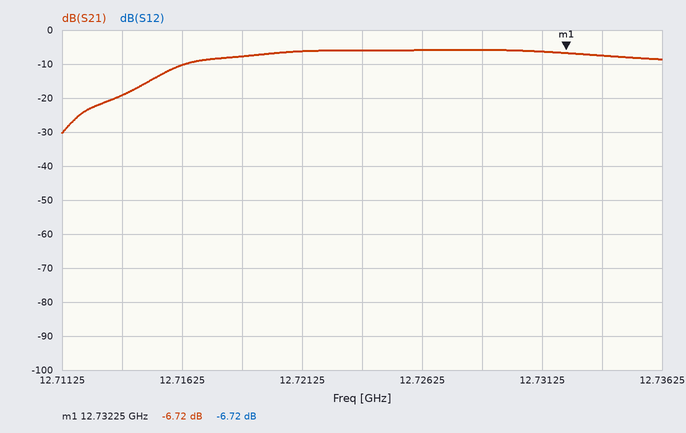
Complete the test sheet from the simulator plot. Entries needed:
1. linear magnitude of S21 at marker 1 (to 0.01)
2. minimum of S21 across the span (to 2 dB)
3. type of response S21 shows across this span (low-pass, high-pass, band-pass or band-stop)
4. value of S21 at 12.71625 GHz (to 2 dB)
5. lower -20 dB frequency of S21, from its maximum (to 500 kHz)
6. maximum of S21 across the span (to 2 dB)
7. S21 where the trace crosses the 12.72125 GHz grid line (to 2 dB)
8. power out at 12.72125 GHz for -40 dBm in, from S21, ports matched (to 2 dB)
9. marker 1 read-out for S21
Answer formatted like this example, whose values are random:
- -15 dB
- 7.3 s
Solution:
- 0.46
- -30 dB
- high-pass
- -10 dB
- 12.7120 GHz
- -6 dB
- -6 dB
- -46 dBm
- -6.72 dB
